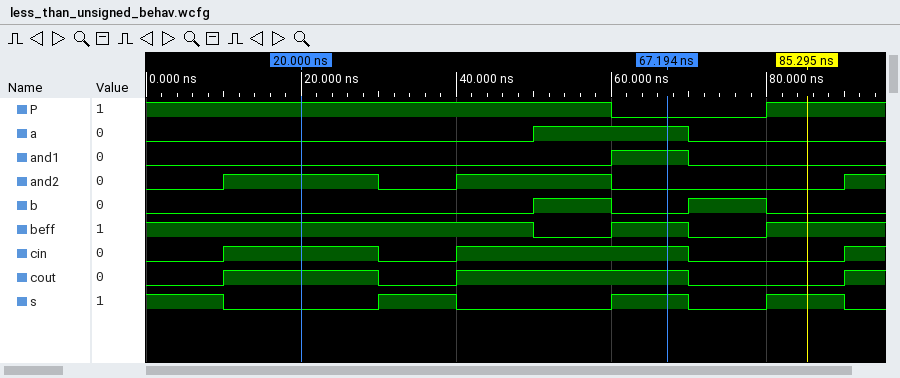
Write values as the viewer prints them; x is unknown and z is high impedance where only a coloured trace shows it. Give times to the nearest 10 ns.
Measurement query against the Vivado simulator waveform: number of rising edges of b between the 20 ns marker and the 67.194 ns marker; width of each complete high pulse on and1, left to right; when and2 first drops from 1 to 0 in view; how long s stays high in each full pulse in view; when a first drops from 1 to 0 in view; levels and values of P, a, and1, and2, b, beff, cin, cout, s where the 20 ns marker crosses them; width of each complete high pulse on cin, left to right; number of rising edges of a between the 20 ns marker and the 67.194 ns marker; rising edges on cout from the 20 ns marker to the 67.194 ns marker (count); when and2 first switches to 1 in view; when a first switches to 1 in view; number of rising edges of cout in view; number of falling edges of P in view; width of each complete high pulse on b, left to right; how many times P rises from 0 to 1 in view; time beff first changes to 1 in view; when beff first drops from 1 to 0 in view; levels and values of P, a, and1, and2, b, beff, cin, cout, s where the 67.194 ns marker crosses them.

1
10 ns
30 ns
10 ns, 10 ns, 10 ns
70 ns
P=1, a=0, and1=0, and2=1, b=0, beff=1, cin=1, cout=1, s=0
20 ns, 30 ns
1
1
10 ns
50 ns
3
1
10 ns, 10 ns
1
60 ns
50 ns
P=0, a=1, and1=1, and2=0, b=0, beff=1, cin=1, cout=1, s=1
